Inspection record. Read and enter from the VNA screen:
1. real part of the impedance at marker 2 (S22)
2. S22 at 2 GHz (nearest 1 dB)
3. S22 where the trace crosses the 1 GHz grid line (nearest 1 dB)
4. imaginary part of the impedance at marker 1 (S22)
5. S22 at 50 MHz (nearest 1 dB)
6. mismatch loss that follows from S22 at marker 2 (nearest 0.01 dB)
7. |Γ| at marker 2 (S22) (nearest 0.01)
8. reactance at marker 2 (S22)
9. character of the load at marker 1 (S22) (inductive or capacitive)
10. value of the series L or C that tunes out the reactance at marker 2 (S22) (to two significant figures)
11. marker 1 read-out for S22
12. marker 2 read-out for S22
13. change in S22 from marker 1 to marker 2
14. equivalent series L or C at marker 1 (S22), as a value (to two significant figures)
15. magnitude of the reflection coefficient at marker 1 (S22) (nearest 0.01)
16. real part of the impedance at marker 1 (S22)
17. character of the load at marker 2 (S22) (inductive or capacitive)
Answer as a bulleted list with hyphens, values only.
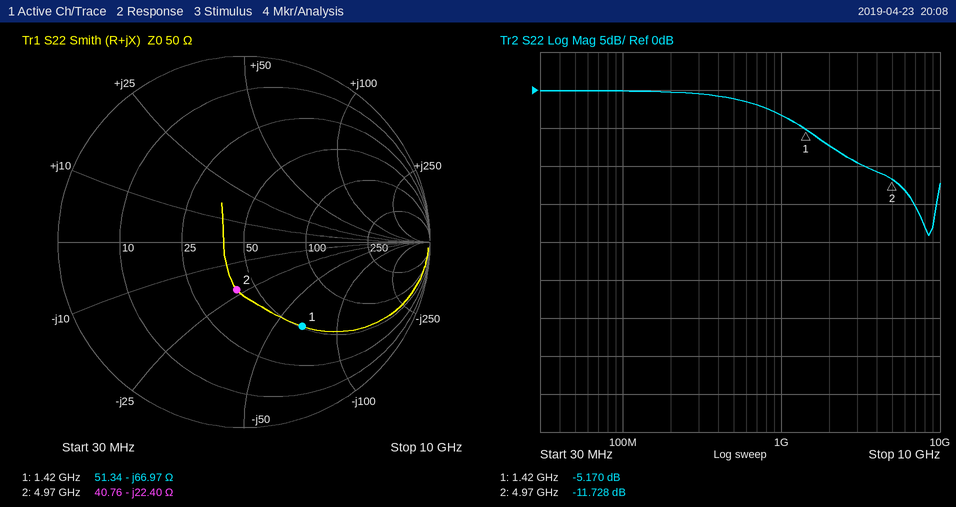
- 40.76 Ω
- -7 dB
- -3 dB
- -66.97 Ω
- 0 dB
- 0.30 dB
- 0.26
- -22.40 Ω
- capacitive
- 720 pH
- -5.170 dB
- -11.728 dB
- -6.558 dB
- 1.7 pF
- 0.55
- 51.34 Ω
- capacitive
